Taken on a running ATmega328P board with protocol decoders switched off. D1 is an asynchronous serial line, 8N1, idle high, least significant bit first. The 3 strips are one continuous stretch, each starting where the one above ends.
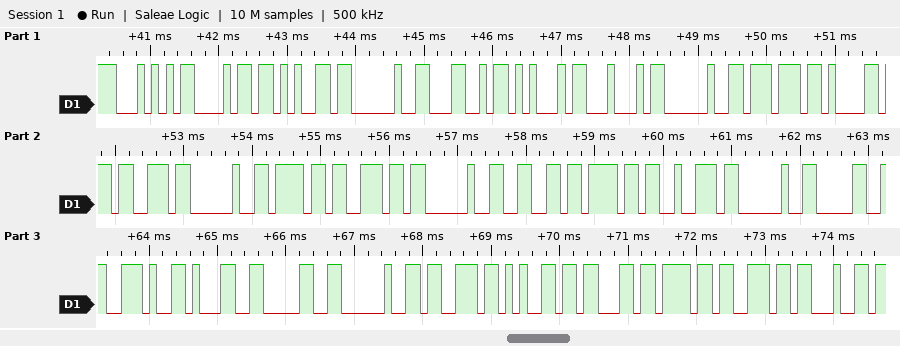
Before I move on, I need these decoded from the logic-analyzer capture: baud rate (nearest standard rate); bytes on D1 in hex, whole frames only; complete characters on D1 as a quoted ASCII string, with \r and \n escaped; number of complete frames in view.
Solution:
9600 baud
54 68 65 20 4C 45 44 20 77 61 73 20 6F 6E 20 66 6F 72 20 30 2E 31 30 20 73 65 63 6F 6E 64
"The LED was on for 0.10 second"
30
